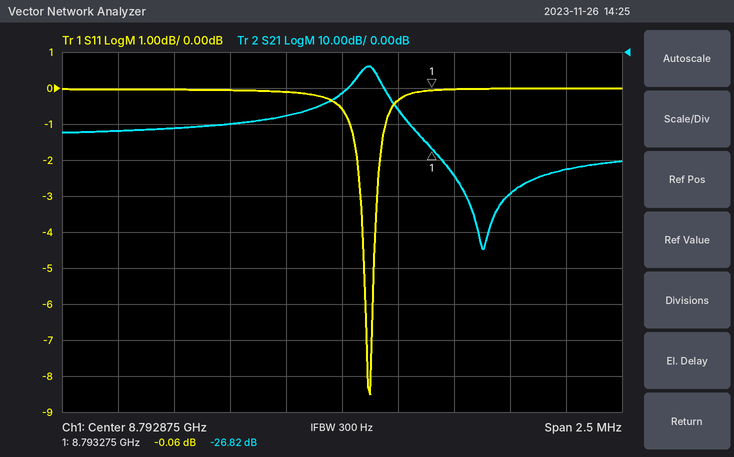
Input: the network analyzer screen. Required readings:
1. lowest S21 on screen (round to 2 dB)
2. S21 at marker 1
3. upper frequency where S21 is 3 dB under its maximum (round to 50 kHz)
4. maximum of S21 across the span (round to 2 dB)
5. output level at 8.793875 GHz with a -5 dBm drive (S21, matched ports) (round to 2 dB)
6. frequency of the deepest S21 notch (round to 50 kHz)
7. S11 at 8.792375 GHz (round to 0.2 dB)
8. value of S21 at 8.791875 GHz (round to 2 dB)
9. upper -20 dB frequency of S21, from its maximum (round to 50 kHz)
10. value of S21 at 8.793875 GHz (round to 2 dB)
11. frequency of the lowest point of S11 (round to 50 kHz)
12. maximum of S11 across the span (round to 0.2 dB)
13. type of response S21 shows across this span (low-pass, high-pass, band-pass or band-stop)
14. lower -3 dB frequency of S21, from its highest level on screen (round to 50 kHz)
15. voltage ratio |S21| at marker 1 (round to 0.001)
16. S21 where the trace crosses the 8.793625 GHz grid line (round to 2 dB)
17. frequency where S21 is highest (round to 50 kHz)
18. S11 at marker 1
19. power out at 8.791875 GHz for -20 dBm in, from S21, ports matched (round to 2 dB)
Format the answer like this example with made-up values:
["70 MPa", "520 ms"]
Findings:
["-54 dB", "-26.82 dB", "8.79305 GHz", "-4 dB", "-38 dBm", "8.79350 GHz", "0.0 dB", "-22 dB", "8.79325 GHz", "-32 dB", "8.79300 GHz", "0.0 dB", "band-pass", "8.79295 GHz", "0.046", "-40 dB", "8.79300 GHz", "-0.06 dB", "-42 dBm"]
